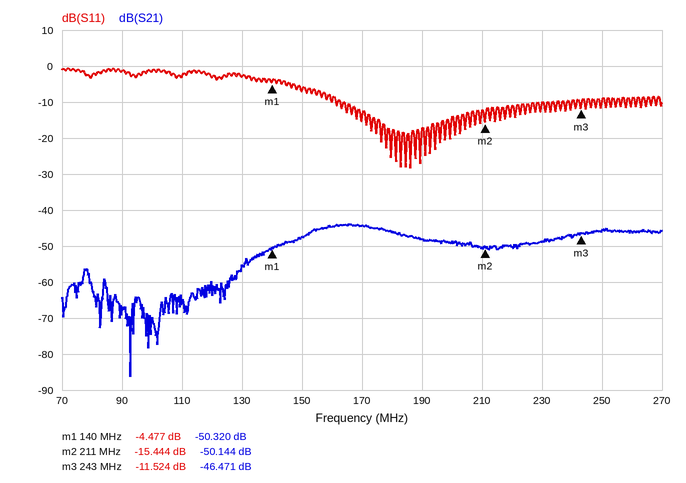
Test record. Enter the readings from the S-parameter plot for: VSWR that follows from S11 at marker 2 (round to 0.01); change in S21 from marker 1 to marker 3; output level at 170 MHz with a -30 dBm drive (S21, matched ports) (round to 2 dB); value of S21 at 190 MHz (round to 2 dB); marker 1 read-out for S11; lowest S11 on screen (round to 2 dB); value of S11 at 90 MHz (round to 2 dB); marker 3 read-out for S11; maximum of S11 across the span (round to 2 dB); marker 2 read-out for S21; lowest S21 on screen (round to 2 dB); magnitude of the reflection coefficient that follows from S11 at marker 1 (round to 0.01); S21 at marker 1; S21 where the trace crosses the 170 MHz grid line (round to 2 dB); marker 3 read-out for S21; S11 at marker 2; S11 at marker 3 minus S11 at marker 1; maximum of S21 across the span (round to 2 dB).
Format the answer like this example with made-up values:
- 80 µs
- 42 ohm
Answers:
- 1.41
- 3.849 dB
- -74 dBm
- -48 dB
- -4.477 dB
- -28 dB
- -2 dB
- -11.524 dB
- 0 dB
- -50.144 dB
- -86 dB
- 0.60
- -50.320 dB
- -44 dB
- -46.471 dB
- -15.444 dB
- -7.047 dB
- -44 dB
